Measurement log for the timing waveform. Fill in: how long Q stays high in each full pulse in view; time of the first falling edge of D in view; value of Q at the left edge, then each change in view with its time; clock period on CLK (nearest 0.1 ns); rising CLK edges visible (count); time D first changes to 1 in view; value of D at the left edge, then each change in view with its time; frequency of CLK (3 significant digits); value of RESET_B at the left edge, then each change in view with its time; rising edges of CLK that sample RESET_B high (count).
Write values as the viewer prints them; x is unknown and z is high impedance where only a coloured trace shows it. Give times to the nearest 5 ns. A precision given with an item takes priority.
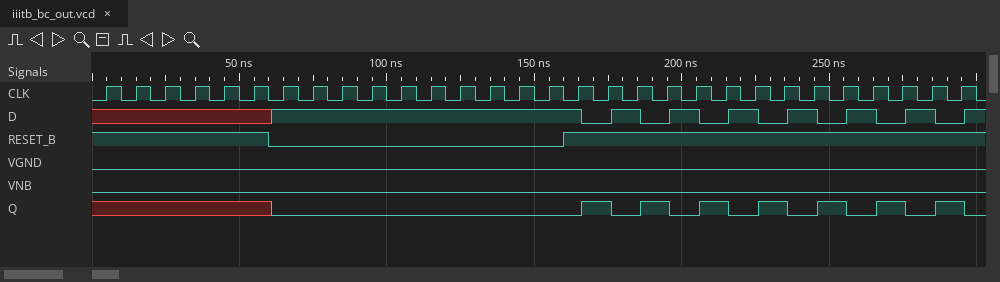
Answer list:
10 ns, 10 ns, 10 ns, 10 ns, 10 ns, 10 ns, 10 ns
165 ns
x, 0 at 60 ns, 1 at 165 ns, 0 at 175 ns, 1 at 185 ns, 0 at 195 ns, 1 at 205 ns, 0 at 215 ns, 1 at 225 ns, 0 at 235 ns, 1 at 245 ns, 0 at 255 ns, 1 at 265 ns, 0 at 275 ns, 1 at 285 ns, 0 at 295 ns
10 ns
30
60 ns
x, 1 at 60 ns, 0 at 165 ns, 1 at 175 ns, 0 at 185 ns, 1 at 195 ns, 0 at 205 ns, 1 at 215 ns, 0 at 225 ns, 1 at 235 ns, 0 at 245 ns, 1 at 255 ns, 0 at 265 ns, 1 at 275 ns, 0 at 285 ns, 1 at 295 ns
100 MHz
1, 0 at 60 ns, 1 at 160 ns
20
